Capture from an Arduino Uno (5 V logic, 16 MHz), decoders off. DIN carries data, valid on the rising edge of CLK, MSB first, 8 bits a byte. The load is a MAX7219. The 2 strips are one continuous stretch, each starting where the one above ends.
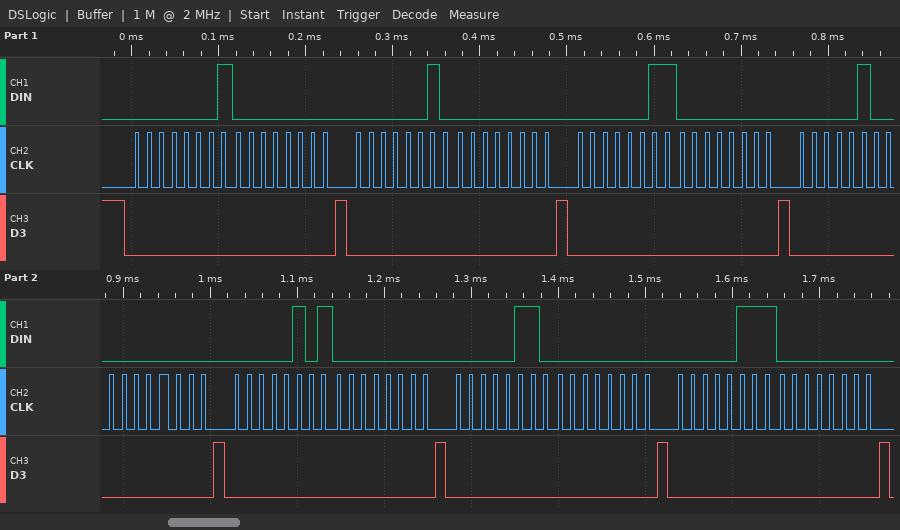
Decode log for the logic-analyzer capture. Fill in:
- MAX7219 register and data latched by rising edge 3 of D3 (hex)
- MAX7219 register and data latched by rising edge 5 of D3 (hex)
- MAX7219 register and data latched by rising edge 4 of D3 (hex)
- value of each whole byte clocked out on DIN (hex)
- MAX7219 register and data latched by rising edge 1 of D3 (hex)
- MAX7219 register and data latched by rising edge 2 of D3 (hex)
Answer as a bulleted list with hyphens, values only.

- register 0x3, data 0x00
- register 0x5, data 0x00
- register 0x4, data 0x00
- 01 00 02 00 03 00 04 00 05 00 06 00 07 00
- register 0x1, data 0x00
- register 0x2, data 0x00
